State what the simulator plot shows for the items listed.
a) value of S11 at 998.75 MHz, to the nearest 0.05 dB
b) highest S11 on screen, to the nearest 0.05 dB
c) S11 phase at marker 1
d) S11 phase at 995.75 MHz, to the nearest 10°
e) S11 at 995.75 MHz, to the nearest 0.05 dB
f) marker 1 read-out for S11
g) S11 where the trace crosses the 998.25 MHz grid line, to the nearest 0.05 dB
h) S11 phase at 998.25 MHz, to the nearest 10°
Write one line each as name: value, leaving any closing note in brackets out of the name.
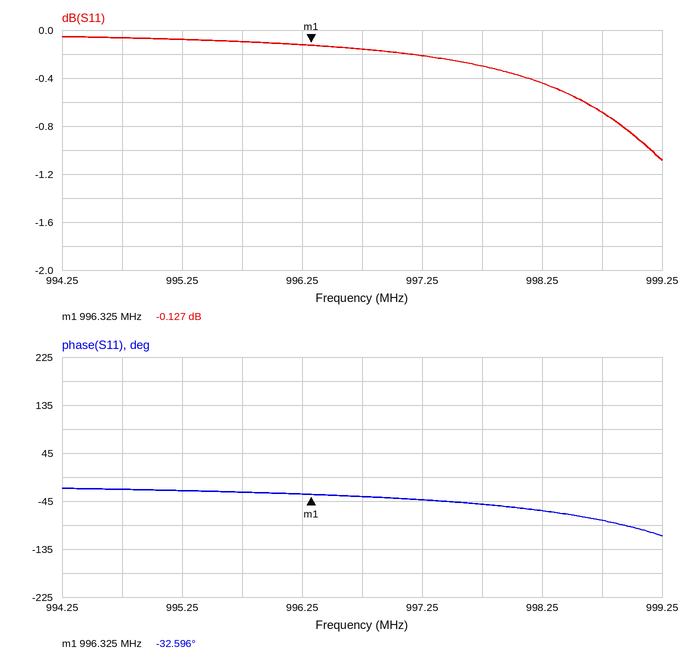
value of S11 at 998.75 MHz, to the nearest 0.05 dB: -0.70 dB
highest S11 on screen, to the nearest 0.05 dB: -0.05 dB
S11 phase at marker 1: -32.596°
S11 phase at 995.75 MHz, to the nearest 10°: -30°
S11 at 995.75 MHz, to the nearest 0.05 dB: -0.10 dB
marker 1 read-out for S11: -0.127 dB
S11 where the trace crosses the 998.25 MHz grid line, to the nearest 0.05 dB: -0.45 dB
S11 phase at 998.25 MHz, to the nearest 10°: -60°
